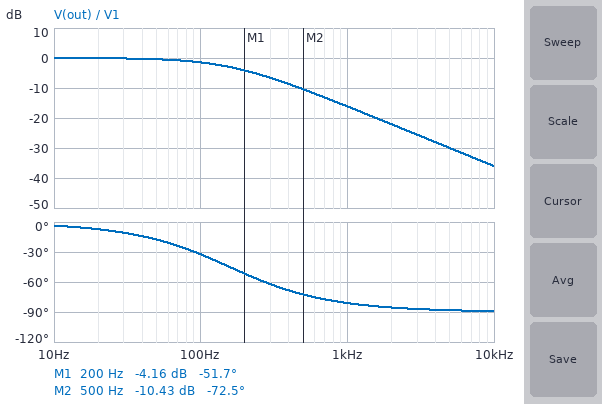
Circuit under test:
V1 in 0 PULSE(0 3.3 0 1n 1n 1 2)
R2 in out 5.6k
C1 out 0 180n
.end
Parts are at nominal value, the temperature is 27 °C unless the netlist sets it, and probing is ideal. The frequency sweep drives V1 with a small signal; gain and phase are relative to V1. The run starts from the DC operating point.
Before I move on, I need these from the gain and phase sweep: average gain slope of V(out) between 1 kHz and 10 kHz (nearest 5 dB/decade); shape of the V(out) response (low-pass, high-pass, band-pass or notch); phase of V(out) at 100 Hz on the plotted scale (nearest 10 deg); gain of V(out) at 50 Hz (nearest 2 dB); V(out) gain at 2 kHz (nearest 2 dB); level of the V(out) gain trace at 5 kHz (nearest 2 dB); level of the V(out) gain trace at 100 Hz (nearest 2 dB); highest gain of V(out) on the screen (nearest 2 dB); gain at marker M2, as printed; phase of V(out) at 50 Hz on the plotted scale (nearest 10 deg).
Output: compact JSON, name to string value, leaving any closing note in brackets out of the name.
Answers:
{"average gain slope of V(out) between 1 kHz and 10 kHz": "-20 dB/decade", "shape of the V(out) response": "low-pass", "phase of V(out) at 100 Hz on the plotted scale": "-30 deg", "gain of V(out) at 50 Hz": "0 dB", "V(out) gain at 2 kHz": "-22 dB", "level of the V(out) gain trace at 5 kHz": "-30 dB", "level of the V(out) gain trace at 100 Hz": "-2 dB", "highest gain of V(out) on the screen": "0 dB", "gain at marker M2, as printed": "-10.43 dB", "phase of V(out) at 50 Hz on the plotted scale": "-20 deg"}
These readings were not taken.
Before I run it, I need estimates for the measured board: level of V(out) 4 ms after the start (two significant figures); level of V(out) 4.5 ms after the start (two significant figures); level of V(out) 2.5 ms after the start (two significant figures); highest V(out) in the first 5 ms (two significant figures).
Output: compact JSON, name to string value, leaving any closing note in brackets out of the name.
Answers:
{"level of V(out) 4 ms after the start": "3.2 V", "level of V(out) 4.5 ms after the start": "3.3 V", "level of V(out) 2.5 ms after the start": "3.0 V", "highest V(out) in the first 5 ms": "3.3 V"}
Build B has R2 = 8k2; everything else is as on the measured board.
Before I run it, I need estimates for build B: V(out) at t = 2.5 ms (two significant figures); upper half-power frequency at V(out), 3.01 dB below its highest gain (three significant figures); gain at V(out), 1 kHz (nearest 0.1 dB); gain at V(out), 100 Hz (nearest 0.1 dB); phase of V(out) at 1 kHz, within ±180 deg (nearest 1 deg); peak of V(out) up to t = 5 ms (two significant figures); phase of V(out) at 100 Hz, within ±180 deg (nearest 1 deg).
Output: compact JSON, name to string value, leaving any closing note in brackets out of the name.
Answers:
{"V(out) at t = 2.5 ms": "2.7 V", "upper half-power frequency at V(out), 3.01 dB below its highest gain": "108 Hz", "gain at V(out), 1 kHz": "-19.4 dB", "gain at V(out), 100 Hz": "-2.7 dB", "phase of V(out) at 1 kHz, within ±180 deg": "-84 deg", "peak of V(out) up to t = 5 ms": "3.2 V", "phase of V(out) at 100 Hz, within ±180 deg": "-43 deg"}
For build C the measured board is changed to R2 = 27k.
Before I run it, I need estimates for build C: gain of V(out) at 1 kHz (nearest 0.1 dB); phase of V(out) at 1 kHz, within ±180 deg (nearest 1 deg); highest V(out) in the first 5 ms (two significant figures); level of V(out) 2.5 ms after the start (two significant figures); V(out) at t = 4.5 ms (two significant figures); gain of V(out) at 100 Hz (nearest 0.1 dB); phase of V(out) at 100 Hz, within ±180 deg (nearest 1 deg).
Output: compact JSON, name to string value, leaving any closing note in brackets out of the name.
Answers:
{"gain of V(out) at 1 kHz": "-29.7 dB", "phase of V(out) at 1 kHz, within ±180 deg": "-88 deg", "highest V(out) in the first 5 ms": "2.1 V", "level of V(out) 2.5 ms after the start": "1.3 V", "V(out) at t = 4.5 ms": "2.0 V", "gain of V(out) at 100 Hz": "-10.1 dB", "phase of V(out) at 100 Hz, within ±180 deg": "-72 deg"}
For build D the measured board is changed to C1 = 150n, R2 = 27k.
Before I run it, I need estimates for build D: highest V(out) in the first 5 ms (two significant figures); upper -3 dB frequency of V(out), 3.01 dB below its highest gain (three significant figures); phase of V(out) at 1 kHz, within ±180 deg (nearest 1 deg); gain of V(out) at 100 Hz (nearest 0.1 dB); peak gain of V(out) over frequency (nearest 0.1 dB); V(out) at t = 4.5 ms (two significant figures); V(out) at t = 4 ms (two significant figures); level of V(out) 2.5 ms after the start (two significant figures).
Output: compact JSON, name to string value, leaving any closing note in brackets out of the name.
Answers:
{"highest V(out) in the first 5 ms": "2.3 V", "upper -3 dB frequency of V(out), 3.01 dB below its highest gain": "39.3 Hz", "phase of V(out) at 1 kHz, within ±180 deg": "-88 deg", "gain of V(out) at 100 Hz": "-8.7 dB", "peak gain of V(out) over frequency": "0 dB", "V(out) at t = 4.5 ms": "2.2 V", "V(out) at t = 4 ms": "2.1 V", "level of V(out) 2.5 ms after the start": "1.5 V"}
